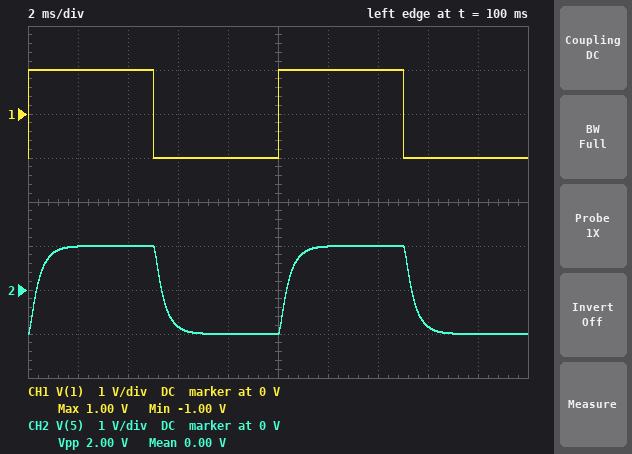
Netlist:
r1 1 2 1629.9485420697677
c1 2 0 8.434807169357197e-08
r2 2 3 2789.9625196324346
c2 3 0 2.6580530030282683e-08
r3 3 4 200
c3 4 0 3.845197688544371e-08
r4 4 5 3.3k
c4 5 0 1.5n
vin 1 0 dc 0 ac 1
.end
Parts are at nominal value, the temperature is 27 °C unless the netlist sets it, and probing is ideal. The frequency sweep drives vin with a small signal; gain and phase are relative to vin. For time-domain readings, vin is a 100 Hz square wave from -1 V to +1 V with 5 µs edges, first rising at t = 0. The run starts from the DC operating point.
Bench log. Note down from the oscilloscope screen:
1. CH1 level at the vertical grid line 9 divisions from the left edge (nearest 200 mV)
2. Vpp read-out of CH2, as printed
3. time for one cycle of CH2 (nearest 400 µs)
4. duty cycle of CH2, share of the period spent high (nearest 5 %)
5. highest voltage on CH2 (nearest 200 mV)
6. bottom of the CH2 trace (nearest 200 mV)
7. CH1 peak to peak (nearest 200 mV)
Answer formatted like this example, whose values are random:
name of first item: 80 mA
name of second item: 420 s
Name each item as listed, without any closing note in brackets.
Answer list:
CH1 level at the vertical grid line 9 divisions from the left edge: -1.0 V
Vpp read-out of CH2, as printed: 2.00 V
time for one cycle of CH2: 10.0 ms
duty cycle of CH2, share of the period spent high: 50 %
highest voltage on CH2: 1.0 V
bottom of the CH2 trace: -1.0 V
CH1 peak to peak: 2.0 V
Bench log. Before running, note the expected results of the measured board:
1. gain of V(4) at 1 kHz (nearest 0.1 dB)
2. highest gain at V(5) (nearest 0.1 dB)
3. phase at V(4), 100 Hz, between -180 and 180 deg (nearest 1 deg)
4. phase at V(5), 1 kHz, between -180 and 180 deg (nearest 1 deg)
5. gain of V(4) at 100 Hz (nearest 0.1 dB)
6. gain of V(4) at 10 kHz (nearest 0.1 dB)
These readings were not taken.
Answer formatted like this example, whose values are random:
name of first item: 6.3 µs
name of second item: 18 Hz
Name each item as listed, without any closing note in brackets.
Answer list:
gain of V(4) at 1 kHz: -8.8 dB
highest gain at V(5): 0 dB
phase at V(4), 100 Hz, between -180 and 180 deg: -16 deg
phase at V(5), 1 kHz, between -180 and 180 deg: -94 deg
gain of V(4) at 100 Hz: -0.2 dB
gain of V(4) at 10 kHz: -40.7 dB
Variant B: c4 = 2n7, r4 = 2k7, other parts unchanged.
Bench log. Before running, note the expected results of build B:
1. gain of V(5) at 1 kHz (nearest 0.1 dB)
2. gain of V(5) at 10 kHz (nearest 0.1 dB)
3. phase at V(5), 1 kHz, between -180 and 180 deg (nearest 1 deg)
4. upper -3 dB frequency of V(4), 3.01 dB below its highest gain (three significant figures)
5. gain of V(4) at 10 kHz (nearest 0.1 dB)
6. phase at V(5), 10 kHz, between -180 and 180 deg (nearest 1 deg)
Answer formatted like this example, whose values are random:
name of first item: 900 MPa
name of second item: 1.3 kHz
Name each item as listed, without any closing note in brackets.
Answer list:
gain of V(5) at 1 kHz: -8.9 dB
gain of V(5) at 10 kHz: -41.6 dB
phase at V(5), 1 kHz, between -180 and 180 deg: -95 deg
upper -3 dB frequency of V(4), 3.01 dB below its highest gain: 415 Hz
gain of V(4) at 10 kHz: -40.8 dB
phase at V(5), 10 kHz, between -180 and 180 deg: 160 deg
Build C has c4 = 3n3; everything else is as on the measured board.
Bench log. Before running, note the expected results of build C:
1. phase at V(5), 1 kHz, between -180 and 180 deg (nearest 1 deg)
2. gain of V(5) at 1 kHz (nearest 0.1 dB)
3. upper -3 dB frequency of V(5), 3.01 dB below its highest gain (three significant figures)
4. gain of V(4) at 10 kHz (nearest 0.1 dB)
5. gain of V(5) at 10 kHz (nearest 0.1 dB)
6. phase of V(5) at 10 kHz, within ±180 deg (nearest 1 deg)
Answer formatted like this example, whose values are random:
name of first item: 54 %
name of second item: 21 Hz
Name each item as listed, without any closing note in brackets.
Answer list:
phase at V(5), 1 kHz, between -180 and 180 deg: -96 deg
gain of V(5) at 1 kHz: -9.0 dB
upper -3 dB frequency of V(5), 3.01 dB below its highest gain: 412 Hz
gain of V(4) at 10 kHz: -40.8 dB
gain of V(5) at 10 kHz: -42.5 dB
phase of V(5) at 10 kHz, within ±180 deg: 151 deg
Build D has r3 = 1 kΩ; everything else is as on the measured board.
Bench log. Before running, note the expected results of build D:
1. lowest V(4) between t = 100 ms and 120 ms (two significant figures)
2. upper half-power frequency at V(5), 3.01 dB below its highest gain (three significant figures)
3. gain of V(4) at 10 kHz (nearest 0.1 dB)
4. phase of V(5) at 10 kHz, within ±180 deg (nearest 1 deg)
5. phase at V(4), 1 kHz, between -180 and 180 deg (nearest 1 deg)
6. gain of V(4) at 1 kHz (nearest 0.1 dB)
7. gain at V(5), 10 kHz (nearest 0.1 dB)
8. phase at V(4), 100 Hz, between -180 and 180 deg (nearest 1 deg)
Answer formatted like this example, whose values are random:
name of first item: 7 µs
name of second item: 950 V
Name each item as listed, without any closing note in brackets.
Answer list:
lowest V(4) between t = 100 ms and 120 ms: -1.0 V
upper half-power frequency at V(5), 3.01 dB below its highest gain: 402 Hz
gain of V(4) at 10 kHz: -43.9 dB
phase of V(5) at 10 kHz, within ±180 deg: 136 deg
phase at V(4), 1 kHz, between -180 and 180 deg: -98 deg
gain of V(4) at 1 kHz: -9.2 dB
gain at V(5), 10 kHz: -44.3 dB
phase at V(4), 100 Hz, between -180 and 180 deg: -17 deg
